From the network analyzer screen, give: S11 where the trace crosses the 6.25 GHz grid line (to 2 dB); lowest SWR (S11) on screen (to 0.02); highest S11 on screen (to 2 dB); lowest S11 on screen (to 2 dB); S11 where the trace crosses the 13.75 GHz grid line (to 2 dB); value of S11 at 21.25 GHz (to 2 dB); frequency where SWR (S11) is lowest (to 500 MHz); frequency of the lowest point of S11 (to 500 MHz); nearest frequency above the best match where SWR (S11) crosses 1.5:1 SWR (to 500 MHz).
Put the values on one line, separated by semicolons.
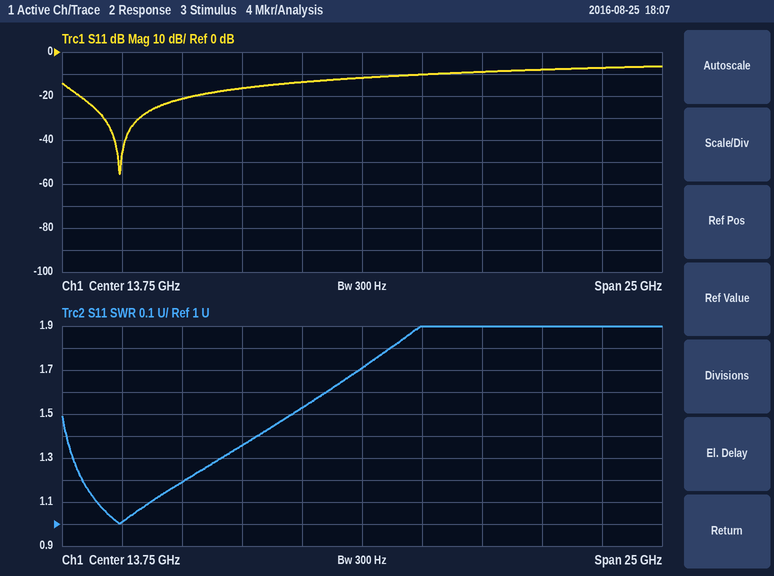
-22 dB; 1.00; -6 dB; -56 dB; -12 dB; -8 dB; 3.5 GHz; 3.5 GHz; 11.0 GHz
